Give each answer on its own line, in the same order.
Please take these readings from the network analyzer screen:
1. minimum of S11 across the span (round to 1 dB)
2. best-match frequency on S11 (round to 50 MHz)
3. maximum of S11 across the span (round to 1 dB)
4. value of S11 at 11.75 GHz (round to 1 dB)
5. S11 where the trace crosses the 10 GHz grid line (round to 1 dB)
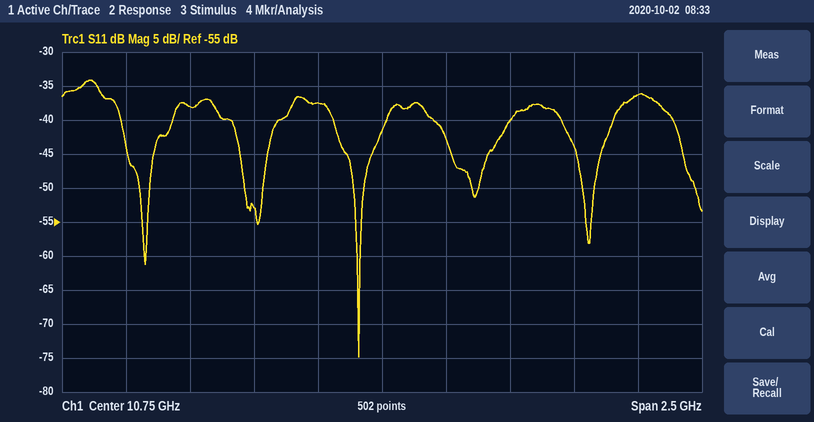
-75 dB
10.65 GHz
-34 dB
-36 dB
-38 dB
